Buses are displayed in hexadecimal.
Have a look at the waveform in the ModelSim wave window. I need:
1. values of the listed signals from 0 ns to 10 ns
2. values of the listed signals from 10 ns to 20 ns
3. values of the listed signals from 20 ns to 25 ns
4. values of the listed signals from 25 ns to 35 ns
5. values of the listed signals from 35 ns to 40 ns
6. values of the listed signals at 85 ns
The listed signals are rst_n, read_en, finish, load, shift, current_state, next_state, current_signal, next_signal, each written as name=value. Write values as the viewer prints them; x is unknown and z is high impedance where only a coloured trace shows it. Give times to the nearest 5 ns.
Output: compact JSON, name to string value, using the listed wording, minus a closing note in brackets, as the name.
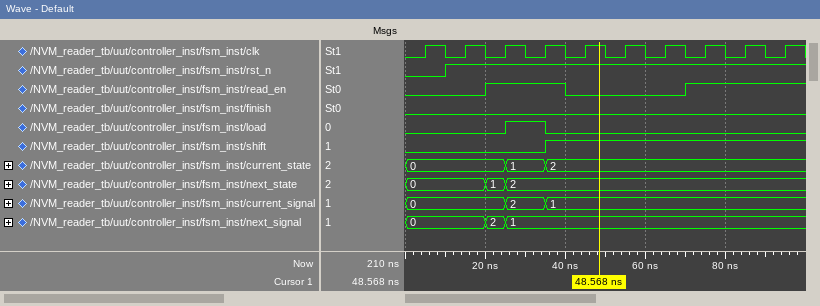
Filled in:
{"values of the listed signals from 0 ns to 10 ns": "rst_n=0, read_en=0, finish=0, load=0, shift=0, current_state=0, next_state=0, current_signal=0, next_signal=0", "values of the listed signals from 10 ns to 20 ns": "rst_n=1, read_en=0, finish=0, load=0, shift=0, current_state=0, next_state=0, current_signal=0, next_signal=0", "values of the listed signals from 20 ns to 25 ns": "rst_n=1, read_en=1, finish=0, load=0, shift=0, current_state=0, next_state=1, current_signal=0, next_signal=2", "values of the listed signals from 25 ns to 35 ns": "rst_n=1, read_en=1, finish=0, load=1, shift=0, current_state=1, next_state=2, current_signal=2, next_signal=1", "values of the listed signals from 35 ns to 40 ns": "rst_n=1, read_en=1, finish=0, load=0, shift=1, current_state=2, next_state=2, current_signal=1, next_signal=1", "values of the listed signals at 85 ns": "rst_n=1, read_en=1, finish=0, load=0, shift=1, current_state=2, next_state=2, current_signal=1, next_signal=1"}
